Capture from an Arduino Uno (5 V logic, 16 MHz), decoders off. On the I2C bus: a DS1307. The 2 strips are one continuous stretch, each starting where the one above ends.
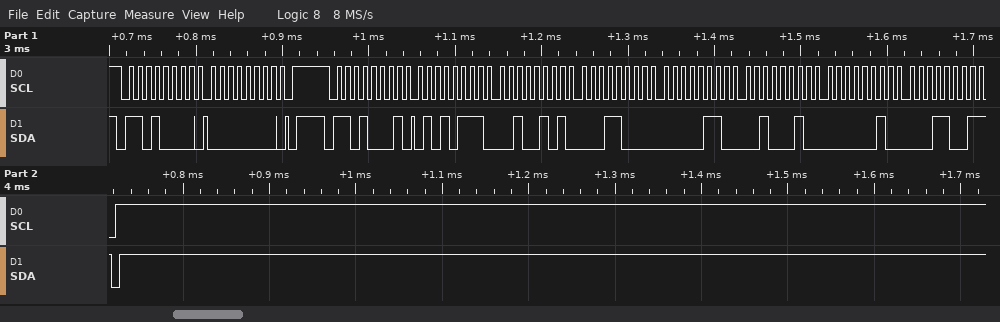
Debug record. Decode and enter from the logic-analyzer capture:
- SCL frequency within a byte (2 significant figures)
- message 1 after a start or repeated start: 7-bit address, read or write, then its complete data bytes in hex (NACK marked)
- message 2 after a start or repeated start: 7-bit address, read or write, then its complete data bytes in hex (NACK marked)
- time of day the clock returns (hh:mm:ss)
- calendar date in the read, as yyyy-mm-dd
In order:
100 kHz
0x68 write: 00
0x68 read: 57 25 18 06 22 02 19 NACK
18:25:57
2019-02-22
